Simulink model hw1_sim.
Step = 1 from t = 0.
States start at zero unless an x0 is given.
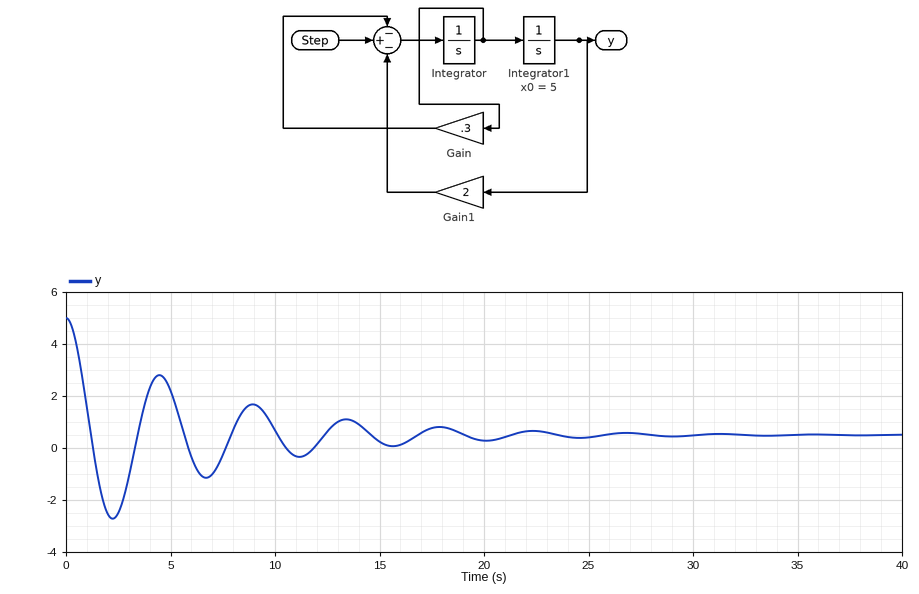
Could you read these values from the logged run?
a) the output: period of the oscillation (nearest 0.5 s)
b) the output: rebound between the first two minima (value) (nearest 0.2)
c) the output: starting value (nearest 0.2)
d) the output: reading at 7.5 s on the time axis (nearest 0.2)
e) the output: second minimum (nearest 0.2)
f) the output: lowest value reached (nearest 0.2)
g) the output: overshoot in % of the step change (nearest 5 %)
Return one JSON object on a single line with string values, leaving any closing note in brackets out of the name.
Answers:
{"the output: period of the oscillation": "4.5 s", "the output: rebound between the first two minima (value)": "2.8", "the output: starting value": "5.0", "the output: reading at 7.5 s on the time axis": "-0.2", "the output: second minimum": "-1.2", "the output: lowest value reached": "-2.8", "the output: overshoot in % of the step change": "70 %"}
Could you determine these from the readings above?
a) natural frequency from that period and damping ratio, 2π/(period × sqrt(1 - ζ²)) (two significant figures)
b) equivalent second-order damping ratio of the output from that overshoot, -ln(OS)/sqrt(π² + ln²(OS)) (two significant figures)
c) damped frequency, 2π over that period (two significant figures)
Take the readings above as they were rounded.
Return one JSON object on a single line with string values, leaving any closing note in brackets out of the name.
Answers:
{"natural frequency from that period and damping ratio, 2π/(period × sqrt(1 - ζ²))": "1.4 rad/s", "equivalent second-order damping ratio of the output from that overshoot, -ln(OS)/sqrt(π² + ln²(OS))": "0.11", "damped frequency, 2π over that period": "1.4 rad/s"}
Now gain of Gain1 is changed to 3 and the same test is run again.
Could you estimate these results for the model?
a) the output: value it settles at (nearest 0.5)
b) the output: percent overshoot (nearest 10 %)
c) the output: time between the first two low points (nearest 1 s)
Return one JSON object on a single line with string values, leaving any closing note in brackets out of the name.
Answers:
{"the output: value it settles at": "0.5", "the output: percent overshoot": "80 %", "the output: time between the first two low points": "4 s"}
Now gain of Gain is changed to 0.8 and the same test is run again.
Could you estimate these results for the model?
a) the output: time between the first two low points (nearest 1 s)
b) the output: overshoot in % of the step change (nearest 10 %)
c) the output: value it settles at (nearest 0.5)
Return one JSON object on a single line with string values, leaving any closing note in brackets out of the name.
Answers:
{"the output: time between the first two low points": "5 s", "the output: overshoot in % of the step change": "40 %", "the output: value it settles at": "0.5"}
